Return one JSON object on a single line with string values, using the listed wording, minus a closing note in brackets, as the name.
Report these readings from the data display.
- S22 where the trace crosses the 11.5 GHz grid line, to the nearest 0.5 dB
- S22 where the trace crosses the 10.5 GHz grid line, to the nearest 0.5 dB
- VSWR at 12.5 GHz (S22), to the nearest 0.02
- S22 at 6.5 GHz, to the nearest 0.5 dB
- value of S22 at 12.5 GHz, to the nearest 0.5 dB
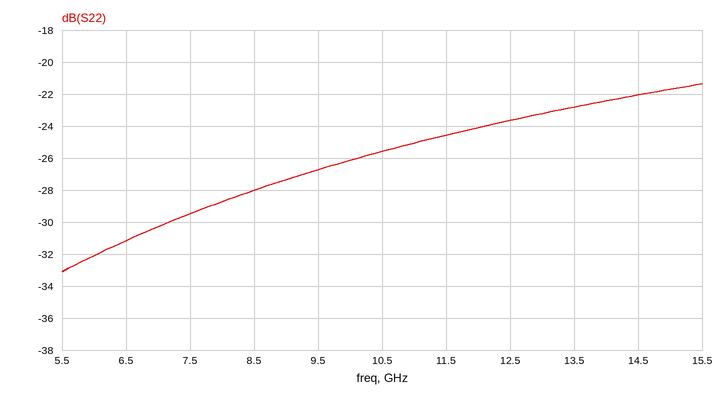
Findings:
{"S22 where the trace crosses the 11.5 GHz grid line, to the nearest 0.5 dB": "-24.5 dB", "S22 where the trace crosses the 10.5 GHz grid line, to the nearest 0.5 dB": "-25.5 dB", "VSWR at 12.5 GHz (S22), to the nearest 0.02": "1.14", "S22 at 6.5 GHz, to the nearest 0.5 dB": "-31.0 dB", "value of S22 at 12.5 GHz, to the nearest 0.5 dB": "-23.5 dB"}
